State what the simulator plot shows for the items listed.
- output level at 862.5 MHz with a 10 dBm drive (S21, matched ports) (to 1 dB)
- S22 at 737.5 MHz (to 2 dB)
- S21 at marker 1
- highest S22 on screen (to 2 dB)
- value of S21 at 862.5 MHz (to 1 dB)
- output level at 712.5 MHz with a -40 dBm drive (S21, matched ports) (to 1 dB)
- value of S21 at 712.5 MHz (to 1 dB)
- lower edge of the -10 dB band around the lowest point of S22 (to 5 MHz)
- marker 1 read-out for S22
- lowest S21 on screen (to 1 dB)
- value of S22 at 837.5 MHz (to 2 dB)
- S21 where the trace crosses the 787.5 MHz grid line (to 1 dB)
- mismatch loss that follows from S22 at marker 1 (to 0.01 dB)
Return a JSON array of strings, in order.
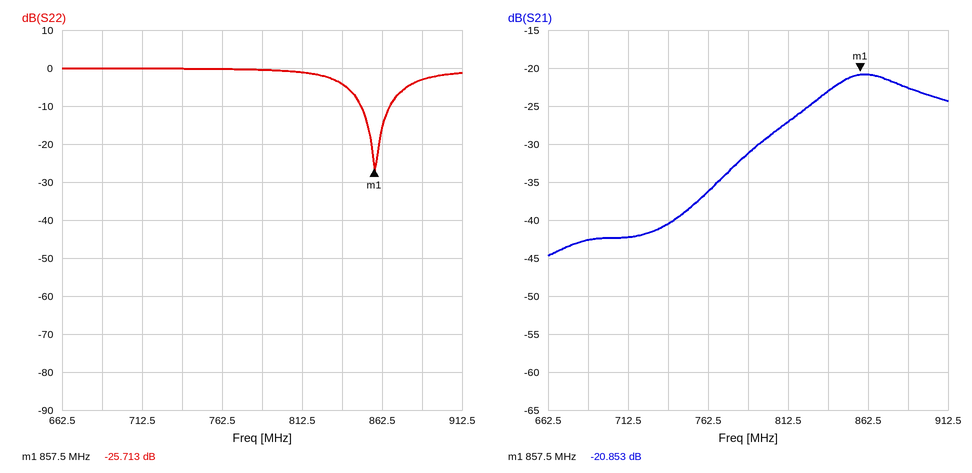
["-11 dBm", "0 dB", "-20.853 dB", "0 dB", "-21 dB", "-82 dBm", "-42 dB", "850 MHz", "-25.713 dB", "-45 dB", "-4 dB", "-31 dB", "0.01 dB"]
